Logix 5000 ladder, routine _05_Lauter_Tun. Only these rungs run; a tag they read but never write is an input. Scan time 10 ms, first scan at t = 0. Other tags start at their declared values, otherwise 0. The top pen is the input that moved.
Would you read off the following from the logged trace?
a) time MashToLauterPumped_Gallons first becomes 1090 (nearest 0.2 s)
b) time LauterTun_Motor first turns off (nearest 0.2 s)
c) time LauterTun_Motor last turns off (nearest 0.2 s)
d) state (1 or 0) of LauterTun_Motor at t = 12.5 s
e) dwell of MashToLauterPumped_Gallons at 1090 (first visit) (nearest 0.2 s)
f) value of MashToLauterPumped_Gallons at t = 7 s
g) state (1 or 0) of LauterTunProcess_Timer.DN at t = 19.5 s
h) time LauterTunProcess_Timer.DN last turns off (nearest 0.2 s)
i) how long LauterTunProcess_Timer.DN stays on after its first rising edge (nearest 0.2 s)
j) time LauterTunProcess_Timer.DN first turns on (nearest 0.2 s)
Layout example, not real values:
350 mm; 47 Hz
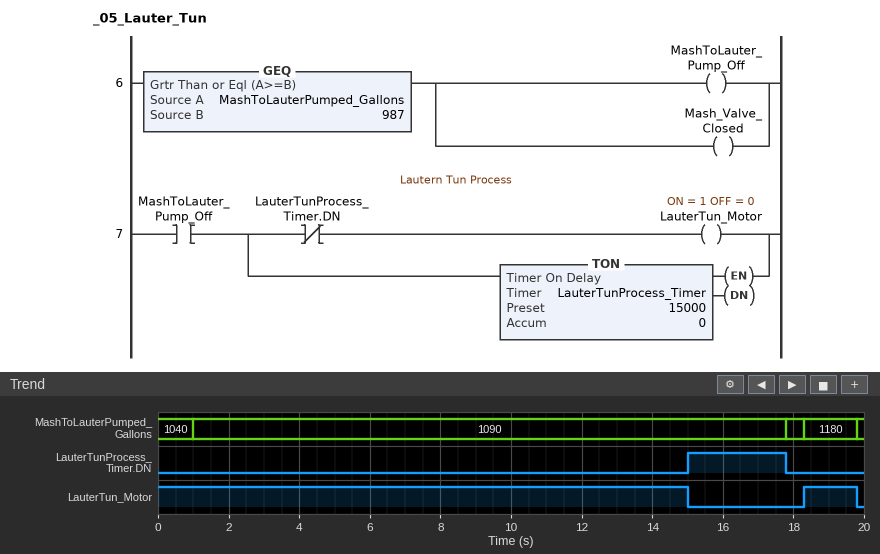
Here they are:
1.0 s; 15.0 s; 19.8 s; 1; 16.8 s; 1090; 0; 17.8 s; 2.8 s; 15.0 s
